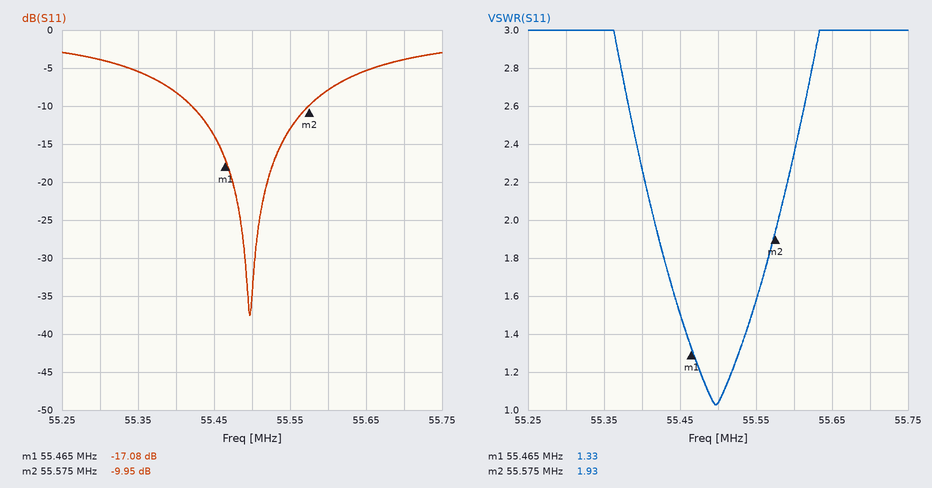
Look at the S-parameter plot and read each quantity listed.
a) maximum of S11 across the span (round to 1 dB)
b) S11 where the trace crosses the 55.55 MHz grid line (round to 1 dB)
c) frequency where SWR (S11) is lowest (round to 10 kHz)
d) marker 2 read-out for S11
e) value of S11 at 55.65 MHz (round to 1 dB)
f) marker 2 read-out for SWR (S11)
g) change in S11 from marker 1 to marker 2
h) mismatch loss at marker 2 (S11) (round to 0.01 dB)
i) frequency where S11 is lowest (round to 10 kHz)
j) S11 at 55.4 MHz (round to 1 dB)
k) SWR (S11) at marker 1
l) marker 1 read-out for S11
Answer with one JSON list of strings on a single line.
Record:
["-3 dB", "-13 dB", "55.50 MHz", "-9.95 dB", "-5 dB", "1.93", "7.13 dB", "0.46 dB", "55.50 MHz", "-8 dB", "1.33", "-17.08 dB"]
